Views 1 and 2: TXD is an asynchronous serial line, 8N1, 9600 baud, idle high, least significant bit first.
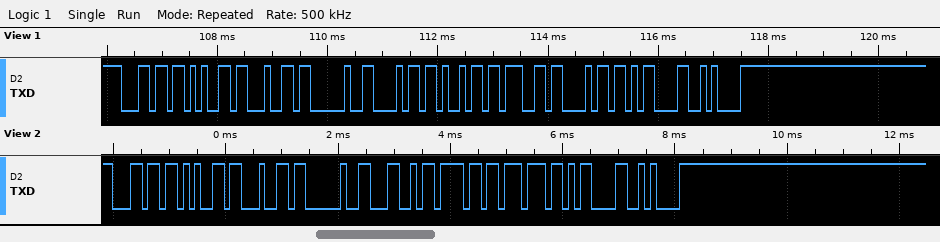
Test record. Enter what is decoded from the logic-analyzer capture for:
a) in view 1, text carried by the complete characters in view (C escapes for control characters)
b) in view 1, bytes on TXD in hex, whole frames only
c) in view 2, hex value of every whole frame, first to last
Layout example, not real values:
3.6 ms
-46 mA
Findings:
"led high\r\n"
6C 65 64 20 68 69 67 68 0D 0A
6C 65 64 20 4C 6F 77 0D 0A
